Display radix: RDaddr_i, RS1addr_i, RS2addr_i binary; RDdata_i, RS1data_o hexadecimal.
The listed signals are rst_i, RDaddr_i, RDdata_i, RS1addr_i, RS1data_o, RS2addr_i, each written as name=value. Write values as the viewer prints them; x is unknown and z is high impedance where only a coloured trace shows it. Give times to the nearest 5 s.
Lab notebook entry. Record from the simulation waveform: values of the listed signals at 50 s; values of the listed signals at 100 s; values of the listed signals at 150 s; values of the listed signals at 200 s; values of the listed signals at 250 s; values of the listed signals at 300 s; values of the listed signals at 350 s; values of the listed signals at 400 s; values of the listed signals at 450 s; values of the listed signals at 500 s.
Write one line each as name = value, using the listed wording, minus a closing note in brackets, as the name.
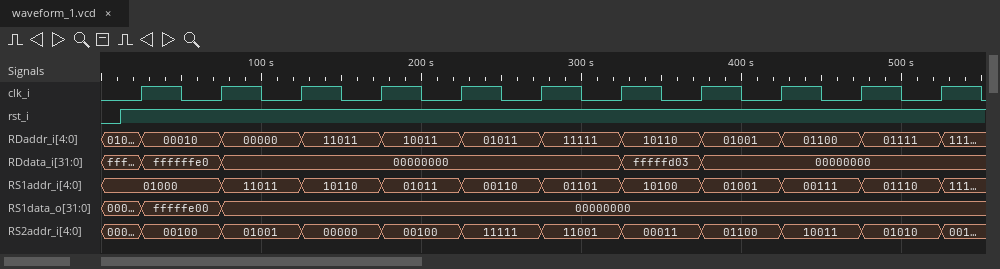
values of the listed signals at 50 s = rst_i=1, RDaddr_i=00010, RDdata_i=ffffffe0, RS1addr_i=01000, RS1data_o=fffffe00, RS2addr_i=00100
values of the listed signals at 100 s = rst_i=1, RDaddr_i=00000, RDdata_i=00000000, RS1addr_i=11011, RS1data_o=00000000, RS2addr_i=01001
values of the listed signals at 150 s = rst_i=1, RDaddr_i=11011, RDdata_i=00000000, RS1addr_i=10110, RS1data_o=00000000, RS2addr_i=00000
values of the listed signals at 200 s = rst_i=1, RDaddr_i=10011, RDdata_i=00000000, RS1addr_i=01011, RS1data_o=00000000, RS2addr_i=00100
values of the listed signals at 250 s = rst_i=1, RDaddr_i=01011, RDdata_i=00000000, RS1addr_i=00110, RS1data_o=00000000, RS2addr_i=11111
values of the listed signals at 300 s = rst_i=1, RDaddr_i=11111, RDdata_i=00000000, RS1addr_i=01101, RS1data_o=00000000, RS2addr_i=11001
values of the listed signals at 350 s = rst_i=1, RDaddr_i=10110, RDdata_i=fffffd03, RS1addr_i=10100, RS1data_o=00000000, RS2addr_i=00011
values of the listed signals at 400 s = rst_i=1, RDaddr_i=01001, RDdata_i=00000000, RS1addr_i=01001, RS1data_o=00000000, RS2addr_i=01100
values of the listed signals at 450 s = rst_i=1, RDaddr_i=01100, RDdata_i=00000000, RS1addr_i=00111, RS1data_o=00000000, RS2addr_i=10011
values of the listed signals at 500 s = rst_i=1, RDaddr_i=01111, RDdata_i=00000000, RS1addr_i=01110, RS1data_o=00000000, RS2addr_i=01010
